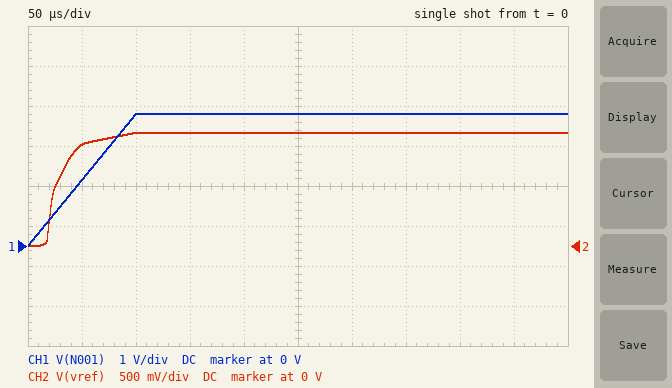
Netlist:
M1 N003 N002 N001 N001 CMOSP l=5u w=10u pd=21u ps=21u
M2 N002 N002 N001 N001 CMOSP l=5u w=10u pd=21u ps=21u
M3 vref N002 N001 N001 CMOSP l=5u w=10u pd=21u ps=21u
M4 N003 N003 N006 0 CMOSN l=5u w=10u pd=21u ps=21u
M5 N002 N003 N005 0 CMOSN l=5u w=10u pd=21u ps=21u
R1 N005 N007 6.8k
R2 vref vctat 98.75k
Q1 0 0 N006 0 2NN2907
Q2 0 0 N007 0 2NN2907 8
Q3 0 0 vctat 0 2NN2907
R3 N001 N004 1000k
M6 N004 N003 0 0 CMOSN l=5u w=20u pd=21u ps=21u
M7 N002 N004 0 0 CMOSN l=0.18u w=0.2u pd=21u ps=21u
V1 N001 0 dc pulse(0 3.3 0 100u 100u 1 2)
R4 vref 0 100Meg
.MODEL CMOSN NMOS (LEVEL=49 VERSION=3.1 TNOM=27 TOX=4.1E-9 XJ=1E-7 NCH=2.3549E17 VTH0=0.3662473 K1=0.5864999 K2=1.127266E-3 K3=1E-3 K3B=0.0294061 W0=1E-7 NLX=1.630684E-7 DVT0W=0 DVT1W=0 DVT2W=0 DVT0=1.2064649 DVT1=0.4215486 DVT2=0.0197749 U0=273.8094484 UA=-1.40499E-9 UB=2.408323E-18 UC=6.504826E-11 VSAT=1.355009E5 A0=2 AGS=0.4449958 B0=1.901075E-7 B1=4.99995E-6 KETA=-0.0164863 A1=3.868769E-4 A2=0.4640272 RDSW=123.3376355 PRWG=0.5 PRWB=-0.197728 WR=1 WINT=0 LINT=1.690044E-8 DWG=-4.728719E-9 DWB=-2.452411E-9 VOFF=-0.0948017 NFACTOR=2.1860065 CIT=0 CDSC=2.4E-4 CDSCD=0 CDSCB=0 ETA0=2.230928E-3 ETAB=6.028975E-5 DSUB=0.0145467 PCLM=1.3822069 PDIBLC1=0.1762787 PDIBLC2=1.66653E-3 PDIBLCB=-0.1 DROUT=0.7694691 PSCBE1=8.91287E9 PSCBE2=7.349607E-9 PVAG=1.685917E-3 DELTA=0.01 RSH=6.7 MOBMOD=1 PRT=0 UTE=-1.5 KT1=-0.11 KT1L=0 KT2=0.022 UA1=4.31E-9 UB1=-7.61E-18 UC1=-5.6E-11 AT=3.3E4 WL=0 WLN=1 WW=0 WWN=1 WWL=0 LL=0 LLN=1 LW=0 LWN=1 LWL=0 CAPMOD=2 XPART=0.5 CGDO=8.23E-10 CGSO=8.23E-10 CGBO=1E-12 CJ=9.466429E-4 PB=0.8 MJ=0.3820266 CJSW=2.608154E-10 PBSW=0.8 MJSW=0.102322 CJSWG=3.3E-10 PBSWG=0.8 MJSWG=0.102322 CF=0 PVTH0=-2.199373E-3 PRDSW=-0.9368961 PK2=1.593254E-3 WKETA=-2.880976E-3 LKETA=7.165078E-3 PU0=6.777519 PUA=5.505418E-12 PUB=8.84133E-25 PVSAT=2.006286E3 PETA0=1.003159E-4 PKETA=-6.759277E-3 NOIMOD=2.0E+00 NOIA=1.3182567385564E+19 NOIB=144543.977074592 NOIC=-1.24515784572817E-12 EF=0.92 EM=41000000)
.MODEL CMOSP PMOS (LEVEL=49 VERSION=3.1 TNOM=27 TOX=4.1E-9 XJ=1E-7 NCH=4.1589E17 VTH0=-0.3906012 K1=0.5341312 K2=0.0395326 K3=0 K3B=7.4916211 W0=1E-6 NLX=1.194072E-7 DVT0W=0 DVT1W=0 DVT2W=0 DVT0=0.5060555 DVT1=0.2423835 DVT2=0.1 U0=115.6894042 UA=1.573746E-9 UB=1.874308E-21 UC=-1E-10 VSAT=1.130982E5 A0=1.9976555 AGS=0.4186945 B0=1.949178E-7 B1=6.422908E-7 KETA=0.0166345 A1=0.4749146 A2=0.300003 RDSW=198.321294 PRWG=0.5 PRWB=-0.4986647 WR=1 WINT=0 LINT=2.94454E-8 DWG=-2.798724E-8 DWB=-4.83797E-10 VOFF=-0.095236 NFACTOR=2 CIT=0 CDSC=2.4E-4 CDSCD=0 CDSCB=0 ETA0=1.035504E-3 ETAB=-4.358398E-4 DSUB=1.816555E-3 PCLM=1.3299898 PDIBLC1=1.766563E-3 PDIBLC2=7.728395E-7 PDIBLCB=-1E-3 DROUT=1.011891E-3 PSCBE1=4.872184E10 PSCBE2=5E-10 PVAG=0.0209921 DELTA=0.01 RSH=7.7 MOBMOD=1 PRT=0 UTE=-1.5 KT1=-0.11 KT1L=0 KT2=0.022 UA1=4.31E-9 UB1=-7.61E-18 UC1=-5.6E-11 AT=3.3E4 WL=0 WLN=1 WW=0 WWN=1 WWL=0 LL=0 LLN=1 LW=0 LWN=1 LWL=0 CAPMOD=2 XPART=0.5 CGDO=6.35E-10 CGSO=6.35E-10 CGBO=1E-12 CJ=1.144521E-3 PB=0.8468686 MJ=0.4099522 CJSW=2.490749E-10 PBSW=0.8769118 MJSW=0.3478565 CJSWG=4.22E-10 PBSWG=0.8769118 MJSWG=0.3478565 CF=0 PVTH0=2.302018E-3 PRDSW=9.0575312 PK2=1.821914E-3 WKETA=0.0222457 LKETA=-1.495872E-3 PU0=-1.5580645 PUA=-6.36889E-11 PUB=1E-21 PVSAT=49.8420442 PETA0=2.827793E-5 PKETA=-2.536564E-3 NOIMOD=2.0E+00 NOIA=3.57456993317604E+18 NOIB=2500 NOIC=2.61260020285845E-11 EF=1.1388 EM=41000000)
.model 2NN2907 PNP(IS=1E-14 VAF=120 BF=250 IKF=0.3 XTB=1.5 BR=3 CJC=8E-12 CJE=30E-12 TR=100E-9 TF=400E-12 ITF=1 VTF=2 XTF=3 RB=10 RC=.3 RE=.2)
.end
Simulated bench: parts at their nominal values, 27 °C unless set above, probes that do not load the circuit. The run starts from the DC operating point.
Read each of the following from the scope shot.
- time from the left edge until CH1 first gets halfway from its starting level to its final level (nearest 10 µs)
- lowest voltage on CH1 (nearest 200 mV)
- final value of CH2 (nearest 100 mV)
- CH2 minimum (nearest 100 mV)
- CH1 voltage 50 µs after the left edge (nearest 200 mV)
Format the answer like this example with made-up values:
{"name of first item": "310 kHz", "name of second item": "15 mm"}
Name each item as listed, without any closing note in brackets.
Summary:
{"time from the left edge until CH1 first gets halfway from its starting level to its final level": "50 µs", "lowest voltage on CH1": "0 V", "final value of CH2": "1.4 V", "CH2 minimum": "0 V", "CH1 voltage 50 µs after the left edge": "1.6 V"}
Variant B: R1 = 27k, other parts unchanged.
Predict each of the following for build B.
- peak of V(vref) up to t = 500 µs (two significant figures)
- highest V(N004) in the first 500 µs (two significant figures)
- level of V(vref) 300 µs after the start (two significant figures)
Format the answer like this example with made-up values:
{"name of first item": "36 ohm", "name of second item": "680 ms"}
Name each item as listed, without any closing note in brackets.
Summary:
{"peak of V(vref) up to t = 500 µs": "1.1 V", "highest V(N004) in the first 500 µs": "410 mV", "level of V(vref) 300 µs after the start": "740 mV"}
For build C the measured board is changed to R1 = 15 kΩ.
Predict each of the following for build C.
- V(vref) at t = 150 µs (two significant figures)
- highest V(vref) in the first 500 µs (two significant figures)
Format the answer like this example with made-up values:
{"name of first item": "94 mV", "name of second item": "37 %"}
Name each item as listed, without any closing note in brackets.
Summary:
{"V(vref) at t = 150 µs": "930 mV", "highest V(vref) in the first 500 µs": "1.1 V"}
